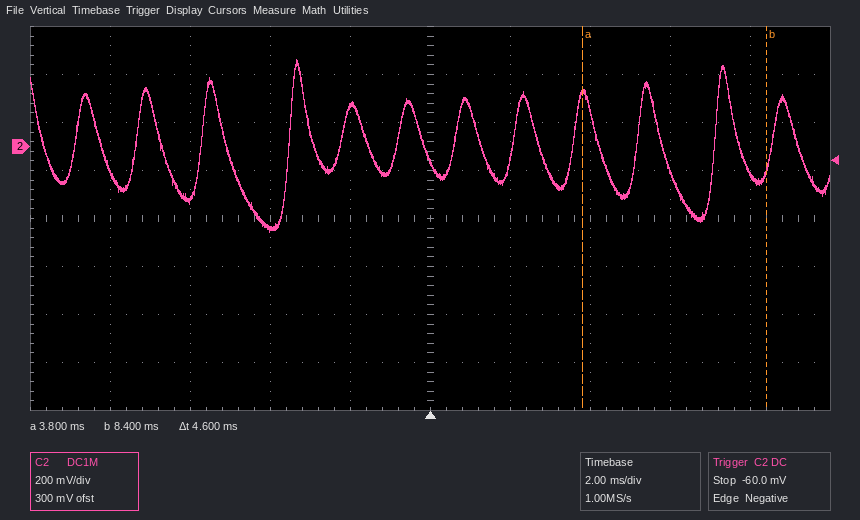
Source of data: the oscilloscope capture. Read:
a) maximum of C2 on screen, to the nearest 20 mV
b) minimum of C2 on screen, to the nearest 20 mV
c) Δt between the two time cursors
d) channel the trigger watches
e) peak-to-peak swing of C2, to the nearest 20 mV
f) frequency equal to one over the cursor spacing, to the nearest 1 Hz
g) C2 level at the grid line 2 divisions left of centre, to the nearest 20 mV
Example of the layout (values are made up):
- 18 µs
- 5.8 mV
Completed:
- 360 mV
- -360 mV
- 4.6 ms
- C2
- 720 mV
- 217 Hz
- -340 mV
